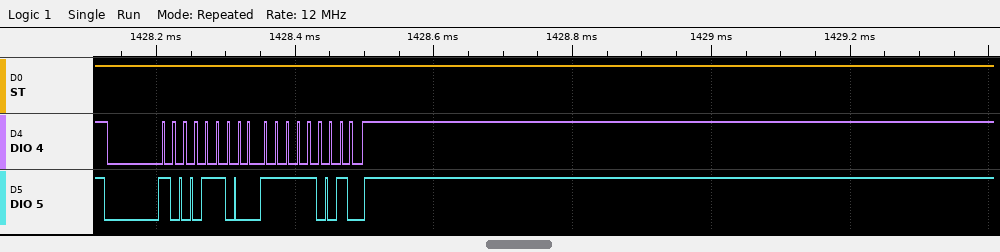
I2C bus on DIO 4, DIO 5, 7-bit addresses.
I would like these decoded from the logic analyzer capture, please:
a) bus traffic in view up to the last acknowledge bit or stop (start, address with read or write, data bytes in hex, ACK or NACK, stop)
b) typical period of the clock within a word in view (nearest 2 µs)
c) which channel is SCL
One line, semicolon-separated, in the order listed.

start, address 46 write ACK, F9 ACK, stop; 16 µs; DIO 4
